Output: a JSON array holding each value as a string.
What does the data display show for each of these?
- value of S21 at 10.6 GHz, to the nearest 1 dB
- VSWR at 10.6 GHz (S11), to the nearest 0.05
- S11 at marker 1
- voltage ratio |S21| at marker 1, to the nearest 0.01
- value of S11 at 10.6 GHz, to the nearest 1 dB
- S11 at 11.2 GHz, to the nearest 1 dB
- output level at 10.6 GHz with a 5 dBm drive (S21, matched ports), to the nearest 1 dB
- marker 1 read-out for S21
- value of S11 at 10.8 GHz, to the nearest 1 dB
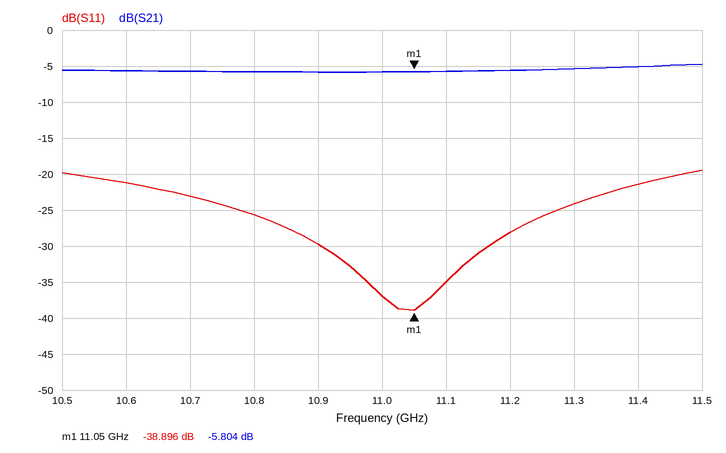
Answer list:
["-6 dB", "1.20", "-38.896 dB", "0.51", "-21 dB", "-28 dB", "-1 dBm", "-5.804 dB", "-26 dB"]
